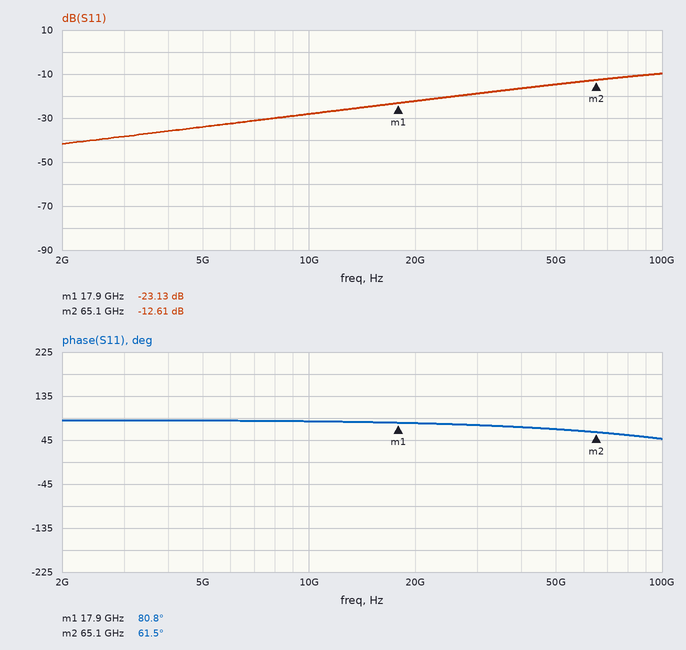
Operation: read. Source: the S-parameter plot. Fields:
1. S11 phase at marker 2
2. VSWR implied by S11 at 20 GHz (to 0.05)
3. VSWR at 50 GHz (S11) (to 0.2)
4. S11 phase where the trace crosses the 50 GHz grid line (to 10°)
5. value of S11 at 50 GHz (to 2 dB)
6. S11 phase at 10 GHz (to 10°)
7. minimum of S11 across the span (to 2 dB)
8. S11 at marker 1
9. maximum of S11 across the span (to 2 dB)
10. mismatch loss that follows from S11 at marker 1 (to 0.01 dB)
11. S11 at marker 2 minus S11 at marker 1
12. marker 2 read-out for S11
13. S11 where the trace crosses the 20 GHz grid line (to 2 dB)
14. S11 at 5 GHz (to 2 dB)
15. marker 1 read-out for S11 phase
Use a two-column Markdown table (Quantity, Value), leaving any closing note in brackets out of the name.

| Quantity | Value |
|---|---|
| S11 phase at marker 2 | 61.5° |
| VSWR implied by S11 at 20 GHz | 1.15 |
| VSWR at 50 GHz (S11) | 1.4 |
| S11 phase where the trace crosses the 50 GHz grid line | 70° |
| value of S11 at 50 GHz | -14 dB |
| S11 phase at 10 GHz | 80° |
| minimum of S11 across the span | -42 dB |
| S11 at marker 1 | -23.13 dB |
| maximum of S11 across the span | -10 dB |
| mismatch loss that follows from S11 at marker 1 | 0.02 dB |
| S11 at marker 2 minus S11 at marker 1 | 10.52 dB |
| marker 2 read-out for S11 | -12.61 dB |
| S11 where the trace crosses the 20 GHz grid line | -22 dB |
| S11 at 5 GHz | -34 dB |
| marker 1 read-out for S11 phase | 80.8° |
